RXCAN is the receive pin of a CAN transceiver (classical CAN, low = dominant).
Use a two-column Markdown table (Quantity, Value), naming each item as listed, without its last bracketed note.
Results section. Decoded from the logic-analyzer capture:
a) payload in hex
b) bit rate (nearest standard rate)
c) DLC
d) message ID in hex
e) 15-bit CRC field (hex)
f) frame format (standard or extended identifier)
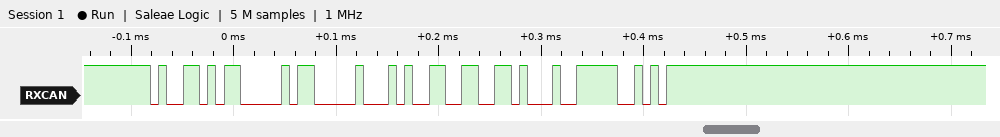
| Quantity | Value |
|---|---|
| payload in hex | 00 A6 66 |
| bit rate | 125 kbit/s |
| DLC | 3 |
| message ID in hex | 0x4D6 |
| 15-bit CRC field | 0x44FA |
| frame format | standard |
